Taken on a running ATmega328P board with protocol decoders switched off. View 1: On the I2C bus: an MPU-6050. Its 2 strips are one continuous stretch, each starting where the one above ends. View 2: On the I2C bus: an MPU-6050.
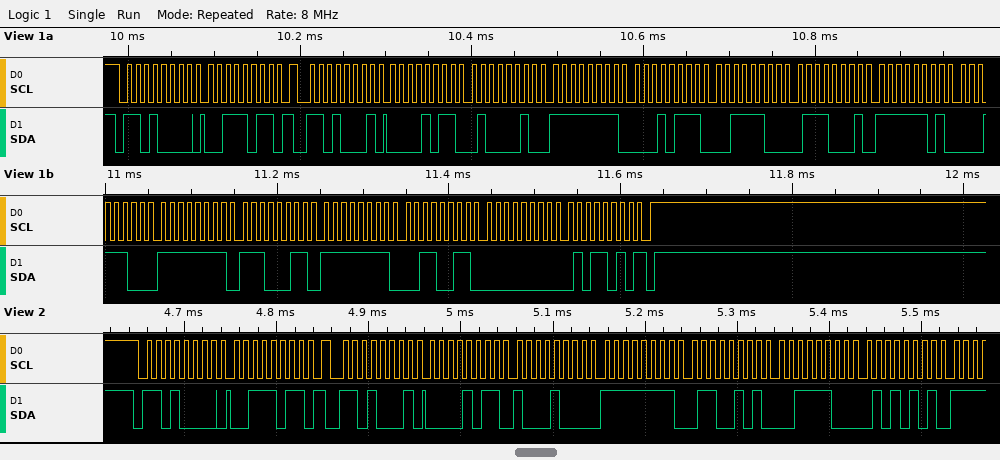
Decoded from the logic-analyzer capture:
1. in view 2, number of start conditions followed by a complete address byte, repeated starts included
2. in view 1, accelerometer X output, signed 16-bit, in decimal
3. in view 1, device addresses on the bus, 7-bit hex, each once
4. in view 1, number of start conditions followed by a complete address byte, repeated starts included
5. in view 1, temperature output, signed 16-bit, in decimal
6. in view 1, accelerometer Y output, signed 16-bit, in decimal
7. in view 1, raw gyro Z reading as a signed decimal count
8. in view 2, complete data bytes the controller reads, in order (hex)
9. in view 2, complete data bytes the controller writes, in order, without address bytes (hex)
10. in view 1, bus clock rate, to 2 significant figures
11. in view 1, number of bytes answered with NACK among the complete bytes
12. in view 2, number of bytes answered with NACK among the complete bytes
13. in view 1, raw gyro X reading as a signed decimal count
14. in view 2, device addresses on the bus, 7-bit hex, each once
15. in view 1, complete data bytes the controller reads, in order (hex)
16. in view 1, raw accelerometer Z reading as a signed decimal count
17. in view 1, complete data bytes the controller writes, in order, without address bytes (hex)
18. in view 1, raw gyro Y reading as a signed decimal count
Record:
2
2882
0x68
2
-740
-233
90
0B 88 FF 65 3C 55
3B
100 kHz
1
0
-29
0x68
0B 42 FF 17 3C 71 FD 1C FF E3 FF 33 00 5A
15473
3B
-205
